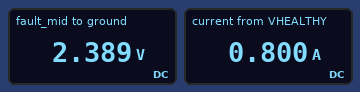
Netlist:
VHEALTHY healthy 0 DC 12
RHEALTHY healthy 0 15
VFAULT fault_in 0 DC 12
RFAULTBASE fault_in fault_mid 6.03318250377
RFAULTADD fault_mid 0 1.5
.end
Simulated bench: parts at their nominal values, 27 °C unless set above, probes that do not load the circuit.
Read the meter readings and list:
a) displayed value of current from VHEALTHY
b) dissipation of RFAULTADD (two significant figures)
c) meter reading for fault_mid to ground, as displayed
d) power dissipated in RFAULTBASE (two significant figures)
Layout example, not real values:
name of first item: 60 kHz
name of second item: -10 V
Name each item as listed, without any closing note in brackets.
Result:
displayed value of current from VHEALTHY: 0.800 A
dissipation of RFAULTADD: 3.8 W
meter reading for fault_mid to ground, as displayed: 2.389 V
power dissipated in RFAULTBASE: 15 W
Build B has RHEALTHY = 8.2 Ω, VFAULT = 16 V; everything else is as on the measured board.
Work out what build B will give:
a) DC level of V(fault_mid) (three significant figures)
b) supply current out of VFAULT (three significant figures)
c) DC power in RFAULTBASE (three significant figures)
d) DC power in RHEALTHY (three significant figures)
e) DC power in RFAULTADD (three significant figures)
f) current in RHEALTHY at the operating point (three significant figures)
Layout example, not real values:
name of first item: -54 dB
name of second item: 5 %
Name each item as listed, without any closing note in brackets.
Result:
DC level of V(fault_mid): 3.19 V
supply current out of VFAULT: 2.12 A
DC power in RFAULTBASE: 27.2 W
DC power in RHEALTHY: 17.6 W
DC power in RFAULTADD: 6.77 W
current in RHEALTHY at the operating point: 1.46 A
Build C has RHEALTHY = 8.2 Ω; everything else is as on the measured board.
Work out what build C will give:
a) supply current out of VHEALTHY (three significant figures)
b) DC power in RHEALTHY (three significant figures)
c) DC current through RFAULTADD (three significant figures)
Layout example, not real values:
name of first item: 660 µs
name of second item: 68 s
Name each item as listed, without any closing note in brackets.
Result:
supply current out of VHEALTHY: 1.46 A
DC power in RHEALTHY: 17.6 W
DC current through RFAULTADD: 1.59 A
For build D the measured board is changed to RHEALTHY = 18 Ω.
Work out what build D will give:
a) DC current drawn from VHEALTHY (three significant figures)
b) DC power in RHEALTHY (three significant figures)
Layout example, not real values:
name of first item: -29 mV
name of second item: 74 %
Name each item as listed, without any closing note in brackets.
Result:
DC current drawn from VHEALTHY: 667 mA
DC power in RHEALTHY: 8.00 W
